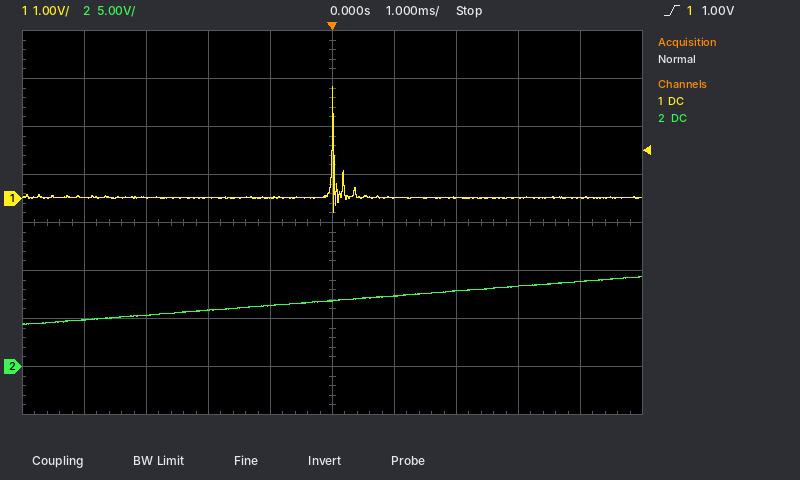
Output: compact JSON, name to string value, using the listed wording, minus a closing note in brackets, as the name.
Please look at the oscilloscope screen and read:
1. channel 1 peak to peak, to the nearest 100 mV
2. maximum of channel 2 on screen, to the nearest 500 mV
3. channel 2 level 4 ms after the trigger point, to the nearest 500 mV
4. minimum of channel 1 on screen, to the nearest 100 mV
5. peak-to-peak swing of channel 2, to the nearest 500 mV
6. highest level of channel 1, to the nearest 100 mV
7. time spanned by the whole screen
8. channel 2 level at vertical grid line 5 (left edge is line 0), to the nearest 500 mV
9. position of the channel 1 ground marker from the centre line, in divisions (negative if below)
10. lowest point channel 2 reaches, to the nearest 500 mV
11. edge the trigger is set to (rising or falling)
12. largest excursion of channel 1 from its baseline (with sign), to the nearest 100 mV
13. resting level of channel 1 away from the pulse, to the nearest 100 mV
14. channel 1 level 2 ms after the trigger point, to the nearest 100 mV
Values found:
{"channel 1 peak to peak, to the nearest 100 mV": "2.6 V", "maximum of channel 2 on screen, to the nearest 500 mV": "9.5 V", "channel 2 level 4 ms after the trigger point, to the nearest 500 mV": "9.0 V", "minimum of channel 1 on screen, to the nearest 100 mV": "-300 mV", "peak-to-peak swing of channel 2, to the nearest 500 mV": "5.0 V", "highest level of channel 1, to the nearest 100 mV": "2.3 V", "time spanned by the whole screen": "10 ms", "channel 2 level at vertical grid line 5 (left edge is line 0), to the nearest 500 mV": "7.0 V", "position of the channel 1 ground marker from the centre line, in divisions": "+0.5 div", "lowest point channel 2 reaches, to the nearest 500 mV": "4.5 V", "edge the trigger is set to": "rising", "largest excursion of channel 1 from its baseline (with sign), to the nearest 100 mV": "+2.3 V", "resting level of channel 1 away from the pulse, to the nearest 100 mV": "0.0 V", "channel 1 level 2 ms after the trigger point, to the nearest 100 mV": "0.0 V"}
